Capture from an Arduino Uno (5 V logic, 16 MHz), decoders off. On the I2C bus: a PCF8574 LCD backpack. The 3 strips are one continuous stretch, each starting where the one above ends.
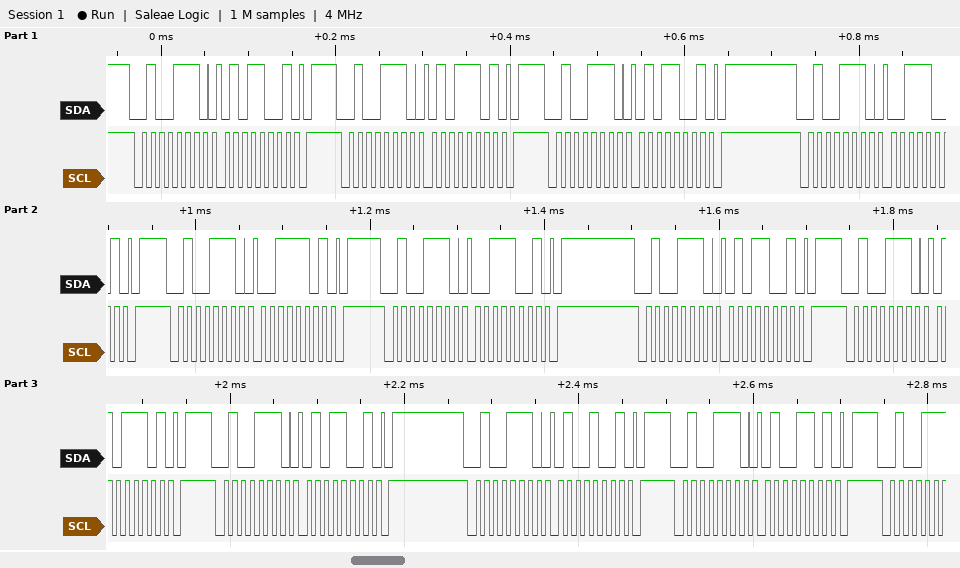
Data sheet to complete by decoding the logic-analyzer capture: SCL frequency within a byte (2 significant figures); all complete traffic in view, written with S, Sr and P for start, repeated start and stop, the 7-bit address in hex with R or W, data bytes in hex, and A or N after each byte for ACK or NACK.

100 kHz
S 27W A 59 A P S 27W A 5D A P S 27W A 59 A P S 27W A 39 A P S 27W A 3D A P S 27W A 39 A P S 27W A 59 A P S 27W A 5D A P S 27W A 59 A P S 27W A 49 A P S 27W A 4D A P
